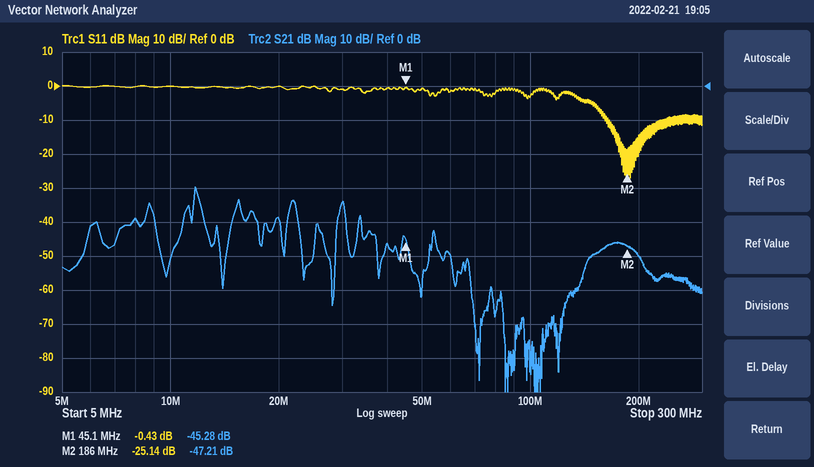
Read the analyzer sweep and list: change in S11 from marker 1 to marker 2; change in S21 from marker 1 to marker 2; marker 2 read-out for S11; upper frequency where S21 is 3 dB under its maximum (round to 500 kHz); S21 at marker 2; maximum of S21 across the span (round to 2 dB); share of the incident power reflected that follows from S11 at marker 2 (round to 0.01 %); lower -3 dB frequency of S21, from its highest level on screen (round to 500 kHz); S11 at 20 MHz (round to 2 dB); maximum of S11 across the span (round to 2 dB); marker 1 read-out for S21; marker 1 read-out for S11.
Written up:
-24.71 dB
-1.93 dB
-25.14 dB
12.0 MHz
-47.21 dB
-30 dB
0.31 %
11.5 MHz
0 dB
0 dB
-45.28 dB
-0.43 dB
